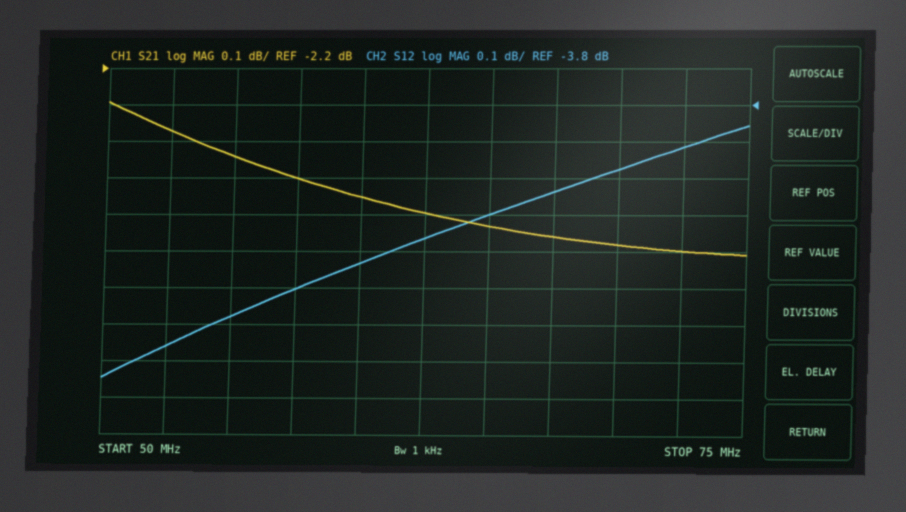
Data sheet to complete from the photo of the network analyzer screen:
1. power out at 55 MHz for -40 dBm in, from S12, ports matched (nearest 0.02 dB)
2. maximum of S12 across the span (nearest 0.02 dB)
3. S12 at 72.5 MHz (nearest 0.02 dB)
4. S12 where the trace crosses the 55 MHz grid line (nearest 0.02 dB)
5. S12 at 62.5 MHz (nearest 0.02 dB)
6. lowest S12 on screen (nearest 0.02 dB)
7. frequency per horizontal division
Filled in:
-44.38 dBm
-3.86 dB
-3.92 dB
-4.38 dB
-4.16 dB
-4.54 dB
2.5 MHz
